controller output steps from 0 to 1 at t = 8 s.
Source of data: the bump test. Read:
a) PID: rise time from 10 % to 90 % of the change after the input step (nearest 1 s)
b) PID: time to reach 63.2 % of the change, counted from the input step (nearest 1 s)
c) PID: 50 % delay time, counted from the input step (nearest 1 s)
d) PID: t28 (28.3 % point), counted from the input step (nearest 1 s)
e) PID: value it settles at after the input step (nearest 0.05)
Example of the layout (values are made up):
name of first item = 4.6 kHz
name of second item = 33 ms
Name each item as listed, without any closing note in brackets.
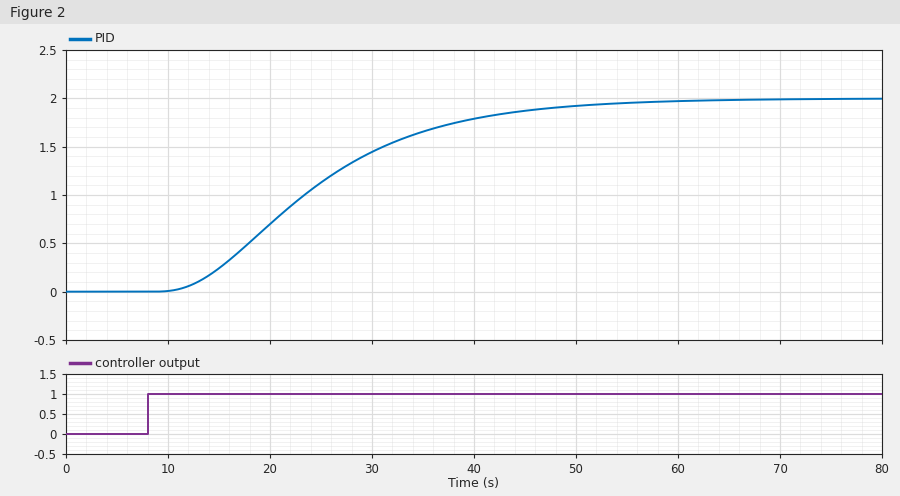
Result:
PID: rise time from 10 % to 90 % of the change after the input step = 26 s
PID: time to reach 63.2 % of the change, counted from the input step = 19 s
PID: 50 % delay time, counted from the input step = 15 s
PID: t28 (28.3 % point), counted from the input step = 11 s
PID: value it settles at after the input step = 2.00
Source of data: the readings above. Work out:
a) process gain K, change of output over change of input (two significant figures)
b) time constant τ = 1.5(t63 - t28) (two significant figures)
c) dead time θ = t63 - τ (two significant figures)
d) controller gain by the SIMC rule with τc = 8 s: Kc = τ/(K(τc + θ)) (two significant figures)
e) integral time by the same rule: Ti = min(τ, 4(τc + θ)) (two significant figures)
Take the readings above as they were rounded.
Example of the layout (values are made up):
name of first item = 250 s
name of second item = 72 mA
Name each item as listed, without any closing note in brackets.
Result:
process gain K, change of output over change of input = 2.0
time constant τ = 1.5(t63 - t28) = 12 s
dead time θ = t63 - τ = 7.0 s
controller gain by the SIMC rule with τc = 8 s: Kc = τ/(K(τc + θ)) = 0.40
integral time by the same rule: Ti = min(τ, 4(τc + θ)) = 12 s
